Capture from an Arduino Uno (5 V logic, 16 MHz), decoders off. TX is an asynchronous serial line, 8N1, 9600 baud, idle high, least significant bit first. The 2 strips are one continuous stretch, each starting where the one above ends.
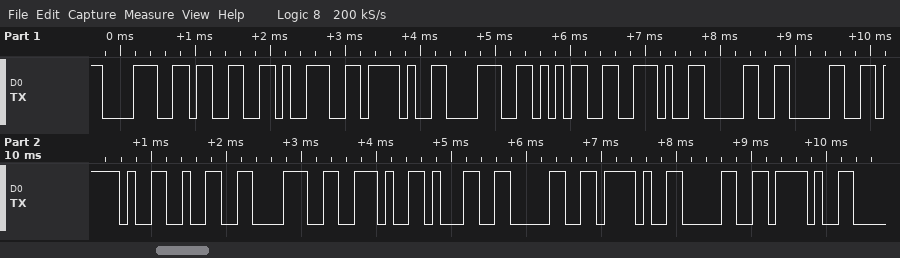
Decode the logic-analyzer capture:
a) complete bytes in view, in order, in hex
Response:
38 33 39 2F 38 35 2E 30 30 2F 32 38 2E 31 30 2F 30 2F
